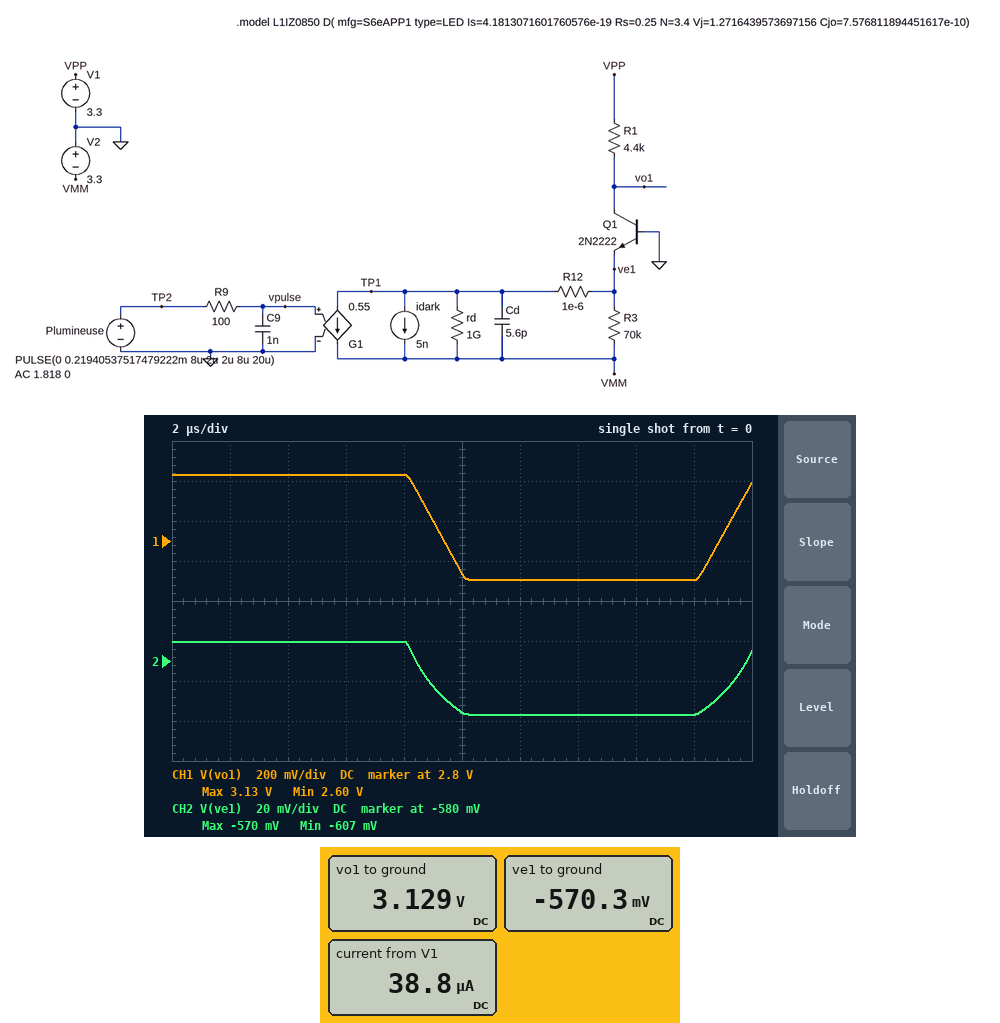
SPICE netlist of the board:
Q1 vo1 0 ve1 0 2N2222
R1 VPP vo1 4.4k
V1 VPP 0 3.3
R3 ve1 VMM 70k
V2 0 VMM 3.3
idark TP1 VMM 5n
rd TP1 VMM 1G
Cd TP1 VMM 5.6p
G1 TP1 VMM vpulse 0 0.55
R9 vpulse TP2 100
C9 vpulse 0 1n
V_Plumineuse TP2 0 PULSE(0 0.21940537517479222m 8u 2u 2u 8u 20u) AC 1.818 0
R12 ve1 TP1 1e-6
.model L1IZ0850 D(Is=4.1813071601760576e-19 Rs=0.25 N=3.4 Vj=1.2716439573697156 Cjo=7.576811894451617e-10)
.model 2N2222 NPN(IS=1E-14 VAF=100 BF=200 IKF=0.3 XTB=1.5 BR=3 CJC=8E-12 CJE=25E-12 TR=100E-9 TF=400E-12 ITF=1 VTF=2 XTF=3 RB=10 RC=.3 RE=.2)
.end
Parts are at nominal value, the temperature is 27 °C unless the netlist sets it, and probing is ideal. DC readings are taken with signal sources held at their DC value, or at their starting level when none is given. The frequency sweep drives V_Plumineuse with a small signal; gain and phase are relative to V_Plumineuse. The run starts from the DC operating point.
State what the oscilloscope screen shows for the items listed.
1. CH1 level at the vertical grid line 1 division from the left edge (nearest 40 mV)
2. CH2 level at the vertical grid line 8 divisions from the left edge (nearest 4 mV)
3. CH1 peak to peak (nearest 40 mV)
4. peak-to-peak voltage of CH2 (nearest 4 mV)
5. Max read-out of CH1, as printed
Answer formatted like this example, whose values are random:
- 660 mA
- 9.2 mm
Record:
- 3.12 V
- -608 mV
- 520 mV
- 36 mV
- 3.13 V
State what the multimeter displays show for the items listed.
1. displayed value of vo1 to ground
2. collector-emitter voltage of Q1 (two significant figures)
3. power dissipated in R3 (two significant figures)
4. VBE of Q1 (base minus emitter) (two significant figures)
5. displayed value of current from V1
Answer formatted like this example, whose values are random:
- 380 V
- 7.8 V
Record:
- 3.129 V
- 3.7 V
- 110 µW
- 570 mV
- 38.8 µA
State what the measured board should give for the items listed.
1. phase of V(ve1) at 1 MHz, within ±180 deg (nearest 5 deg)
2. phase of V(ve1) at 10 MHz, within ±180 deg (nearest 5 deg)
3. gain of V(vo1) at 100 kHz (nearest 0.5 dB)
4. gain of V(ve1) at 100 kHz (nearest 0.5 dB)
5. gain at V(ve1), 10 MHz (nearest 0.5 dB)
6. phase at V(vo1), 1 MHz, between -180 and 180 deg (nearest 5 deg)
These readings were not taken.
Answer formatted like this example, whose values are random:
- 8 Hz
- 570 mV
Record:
- 140 deg
- 40 deg
- 67.5 dB
- 51.0 dB
- 29.0 dB
- 130 deg
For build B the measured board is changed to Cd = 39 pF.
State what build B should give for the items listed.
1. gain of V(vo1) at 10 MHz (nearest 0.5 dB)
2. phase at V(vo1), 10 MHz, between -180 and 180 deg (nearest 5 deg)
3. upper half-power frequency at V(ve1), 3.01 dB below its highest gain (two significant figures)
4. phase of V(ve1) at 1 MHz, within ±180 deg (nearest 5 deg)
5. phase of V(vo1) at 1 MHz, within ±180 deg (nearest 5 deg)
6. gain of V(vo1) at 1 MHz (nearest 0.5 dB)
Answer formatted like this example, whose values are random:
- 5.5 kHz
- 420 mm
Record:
- 37.0 dB
- -25 deg
- 1.3 MHz
- 130 deg
- 125 deg
- 65.5 dB
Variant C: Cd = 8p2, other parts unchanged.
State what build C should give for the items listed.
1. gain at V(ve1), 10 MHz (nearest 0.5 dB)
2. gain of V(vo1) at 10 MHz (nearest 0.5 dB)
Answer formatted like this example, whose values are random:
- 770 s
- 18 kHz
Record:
- 28.5 dB
- 40.5 dB
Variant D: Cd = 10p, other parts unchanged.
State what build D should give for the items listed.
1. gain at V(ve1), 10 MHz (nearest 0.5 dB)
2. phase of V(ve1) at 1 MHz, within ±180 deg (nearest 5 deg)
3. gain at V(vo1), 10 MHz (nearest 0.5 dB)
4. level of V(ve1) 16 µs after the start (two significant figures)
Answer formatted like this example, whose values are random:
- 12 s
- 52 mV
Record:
- 28.5 dB
- 135 deg
- 40.5 dB
- -610 mV
